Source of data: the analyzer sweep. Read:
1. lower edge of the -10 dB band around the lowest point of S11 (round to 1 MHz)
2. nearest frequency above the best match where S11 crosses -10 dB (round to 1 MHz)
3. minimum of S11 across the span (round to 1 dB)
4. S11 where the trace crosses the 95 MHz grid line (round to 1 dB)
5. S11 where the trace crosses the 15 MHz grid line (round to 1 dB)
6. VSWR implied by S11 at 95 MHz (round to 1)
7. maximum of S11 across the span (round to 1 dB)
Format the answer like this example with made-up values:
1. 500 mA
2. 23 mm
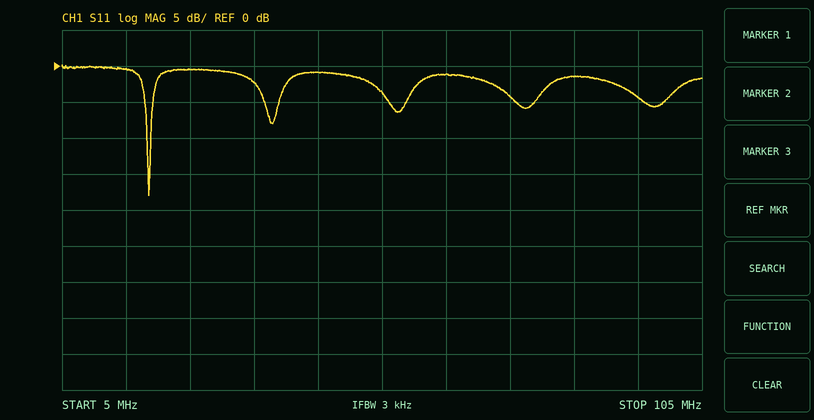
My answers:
1. 18 MHz
2. 19 MHz
3. -18 dB
4. -4 dB
5. 0 dB
6. 4
7. 0 dB
